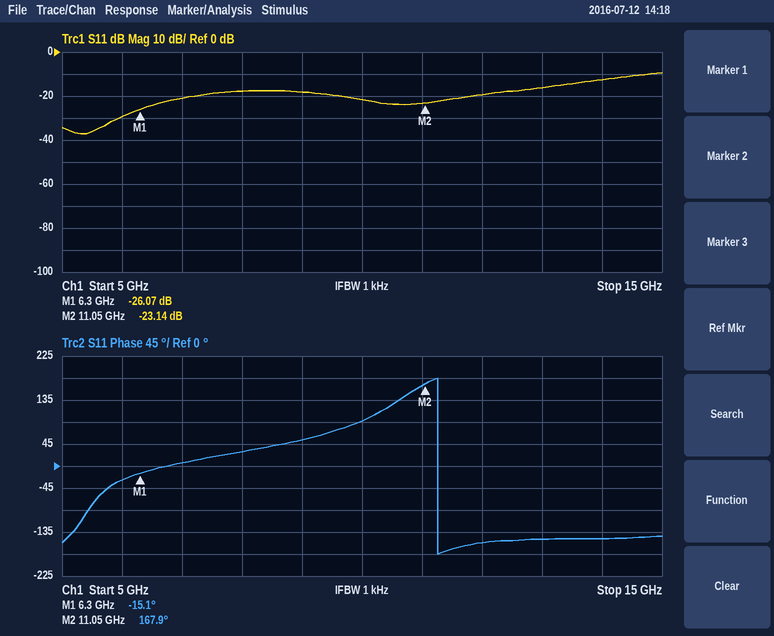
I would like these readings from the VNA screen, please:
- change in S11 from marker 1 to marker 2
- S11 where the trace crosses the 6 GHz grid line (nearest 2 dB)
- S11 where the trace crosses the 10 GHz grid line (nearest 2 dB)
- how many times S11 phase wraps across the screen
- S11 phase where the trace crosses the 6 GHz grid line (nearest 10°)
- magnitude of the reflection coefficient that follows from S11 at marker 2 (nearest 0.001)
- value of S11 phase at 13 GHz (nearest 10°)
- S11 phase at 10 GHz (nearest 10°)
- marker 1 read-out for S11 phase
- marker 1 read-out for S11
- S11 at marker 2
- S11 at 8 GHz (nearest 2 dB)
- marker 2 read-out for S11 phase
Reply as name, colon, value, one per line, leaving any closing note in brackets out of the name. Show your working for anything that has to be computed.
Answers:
change in S11 from marker 1 to marker 2: -23.14 − (-26.07) = 2.93 dB
S11 where the trace crosses the 6 GHz grid line: -30 dB
S11 where the trace crosses the 10 GHz grid line: -22 dB
how many times S11 phase wraps across the screen: 1
S11 phase where the trace crosses the 6 GHz grid line: -30°
magnitude of the reflection coefficient that follows from S11 at marker 2: 10^(-23.14/20) ≈ 0.070
value of S11 phase at 13 GHz: -150°
S11 phase at 10 GHz: 90°
marker 1 read-out for S11 phase: -15.1°
marker 1 read-out for S11: -26.07 dB
S11 at marker 2: -23.14 dB
S11 at 8 GHz: -18 dB
marker 2 read-out for S11 phase: 167.9°
